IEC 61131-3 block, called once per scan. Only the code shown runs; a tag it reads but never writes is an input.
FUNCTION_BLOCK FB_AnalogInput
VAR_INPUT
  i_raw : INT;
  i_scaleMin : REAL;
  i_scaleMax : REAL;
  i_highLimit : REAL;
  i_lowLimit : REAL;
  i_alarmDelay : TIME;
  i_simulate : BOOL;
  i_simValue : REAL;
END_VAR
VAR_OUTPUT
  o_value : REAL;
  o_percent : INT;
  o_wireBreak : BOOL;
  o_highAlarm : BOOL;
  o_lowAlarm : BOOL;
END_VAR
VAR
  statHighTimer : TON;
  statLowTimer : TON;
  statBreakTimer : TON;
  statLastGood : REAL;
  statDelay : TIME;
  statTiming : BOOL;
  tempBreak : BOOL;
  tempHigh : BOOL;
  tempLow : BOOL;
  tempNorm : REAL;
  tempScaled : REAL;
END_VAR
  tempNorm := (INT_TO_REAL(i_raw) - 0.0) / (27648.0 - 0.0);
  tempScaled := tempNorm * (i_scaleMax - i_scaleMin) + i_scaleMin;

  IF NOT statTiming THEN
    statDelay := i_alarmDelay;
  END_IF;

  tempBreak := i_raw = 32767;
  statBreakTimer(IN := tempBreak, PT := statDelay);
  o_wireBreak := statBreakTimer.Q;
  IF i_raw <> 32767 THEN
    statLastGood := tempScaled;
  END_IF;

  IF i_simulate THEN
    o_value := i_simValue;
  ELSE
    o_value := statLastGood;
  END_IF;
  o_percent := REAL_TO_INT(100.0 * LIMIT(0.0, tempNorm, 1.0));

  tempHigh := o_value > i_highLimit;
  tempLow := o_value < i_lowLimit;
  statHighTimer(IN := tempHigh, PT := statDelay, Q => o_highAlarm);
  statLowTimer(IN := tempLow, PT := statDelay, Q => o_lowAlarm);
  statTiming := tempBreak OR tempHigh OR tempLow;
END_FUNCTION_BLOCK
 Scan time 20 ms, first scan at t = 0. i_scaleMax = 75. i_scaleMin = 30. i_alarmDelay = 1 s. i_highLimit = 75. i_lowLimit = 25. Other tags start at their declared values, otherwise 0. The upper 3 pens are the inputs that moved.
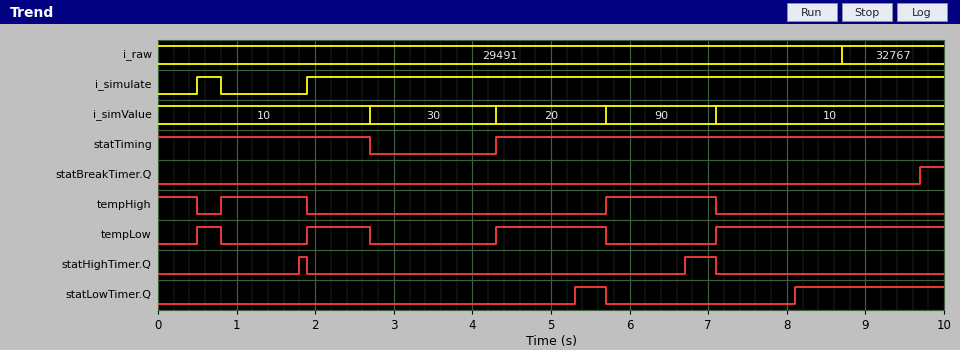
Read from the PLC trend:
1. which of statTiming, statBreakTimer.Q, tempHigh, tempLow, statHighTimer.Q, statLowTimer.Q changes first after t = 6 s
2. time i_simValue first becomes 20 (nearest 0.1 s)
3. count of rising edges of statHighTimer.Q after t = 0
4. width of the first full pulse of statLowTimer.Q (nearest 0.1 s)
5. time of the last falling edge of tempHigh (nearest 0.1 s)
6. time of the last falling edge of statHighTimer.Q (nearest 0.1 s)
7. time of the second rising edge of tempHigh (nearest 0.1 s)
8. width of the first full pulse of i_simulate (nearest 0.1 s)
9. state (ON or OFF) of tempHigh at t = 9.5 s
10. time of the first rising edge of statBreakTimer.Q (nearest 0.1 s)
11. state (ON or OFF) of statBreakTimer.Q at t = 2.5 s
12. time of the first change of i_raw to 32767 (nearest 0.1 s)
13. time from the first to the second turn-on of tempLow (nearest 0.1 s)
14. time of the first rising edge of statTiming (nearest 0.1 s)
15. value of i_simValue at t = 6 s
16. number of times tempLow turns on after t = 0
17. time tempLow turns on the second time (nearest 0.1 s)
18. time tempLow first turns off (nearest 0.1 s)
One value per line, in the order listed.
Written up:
statHighTimer.Q
4.3 s
2
0.4 s
7.1 s
7.1 s
5.7 s
0.3 s
OFF
9.7 s
OFF
8.7 s
1.4 s
4.3 s
90
4
1.9 s
0.8 s
